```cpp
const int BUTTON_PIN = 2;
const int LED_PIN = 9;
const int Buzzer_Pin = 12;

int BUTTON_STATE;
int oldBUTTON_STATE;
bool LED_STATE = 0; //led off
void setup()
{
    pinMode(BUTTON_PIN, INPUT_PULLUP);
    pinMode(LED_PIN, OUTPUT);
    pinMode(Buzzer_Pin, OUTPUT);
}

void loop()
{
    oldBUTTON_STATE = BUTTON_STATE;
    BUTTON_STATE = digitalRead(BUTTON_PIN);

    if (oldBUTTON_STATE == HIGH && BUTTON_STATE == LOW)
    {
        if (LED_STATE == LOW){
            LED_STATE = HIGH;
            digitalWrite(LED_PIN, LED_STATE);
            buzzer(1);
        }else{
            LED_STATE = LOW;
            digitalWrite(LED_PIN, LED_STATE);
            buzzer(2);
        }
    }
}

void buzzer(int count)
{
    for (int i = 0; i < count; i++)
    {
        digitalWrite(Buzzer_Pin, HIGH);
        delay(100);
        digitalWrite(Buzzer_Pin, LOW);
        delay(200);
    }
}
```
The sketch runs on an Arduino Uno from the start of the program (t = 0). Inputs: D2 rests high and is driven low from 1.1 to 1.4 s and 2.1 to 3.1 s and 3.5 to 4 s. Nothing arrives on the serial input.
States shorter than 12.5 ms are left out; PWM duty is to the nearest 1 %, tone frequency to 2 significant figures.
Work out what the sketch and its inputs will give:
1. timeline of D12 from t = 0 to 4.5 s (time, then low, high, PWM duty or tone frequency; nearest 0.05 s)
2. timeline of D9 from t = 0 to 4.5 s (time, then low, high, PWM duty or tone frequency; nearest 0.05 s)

0 s low; 1.1 s high; 1.2 s low; 2.1 s high; 2.2 s low; 2.4 s high; 2.5 s low; 3.5 s high; 3.6 s low
0 s low; 1.1 s high; 2.1 s low; 3.5 s high
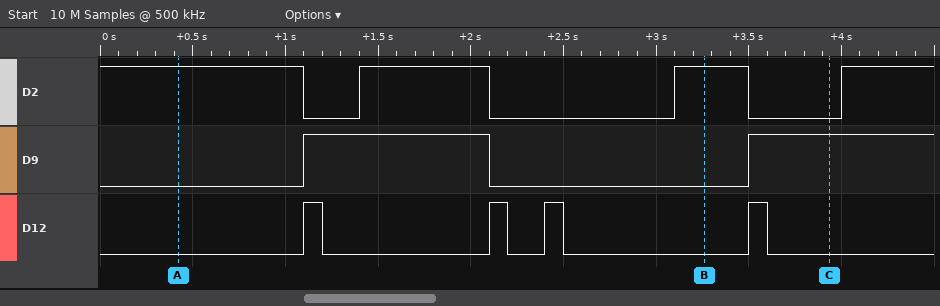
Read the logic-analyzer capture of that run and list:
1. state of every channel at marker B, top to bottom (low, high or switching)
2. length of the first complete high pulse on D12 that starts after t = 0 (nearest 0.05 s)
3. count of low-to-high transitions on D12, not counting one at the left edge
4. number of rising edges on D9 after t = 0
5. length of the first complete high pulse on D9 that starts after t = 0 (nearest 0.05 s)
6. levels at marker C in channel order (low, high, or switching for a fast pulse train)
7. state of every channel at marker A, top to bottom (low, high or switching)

D2 high, D9 low, D12 low
0.10 s
4
2
1.00 s
D2 low, D9 high, D12 low
D2 high, D9 low, D12 low
